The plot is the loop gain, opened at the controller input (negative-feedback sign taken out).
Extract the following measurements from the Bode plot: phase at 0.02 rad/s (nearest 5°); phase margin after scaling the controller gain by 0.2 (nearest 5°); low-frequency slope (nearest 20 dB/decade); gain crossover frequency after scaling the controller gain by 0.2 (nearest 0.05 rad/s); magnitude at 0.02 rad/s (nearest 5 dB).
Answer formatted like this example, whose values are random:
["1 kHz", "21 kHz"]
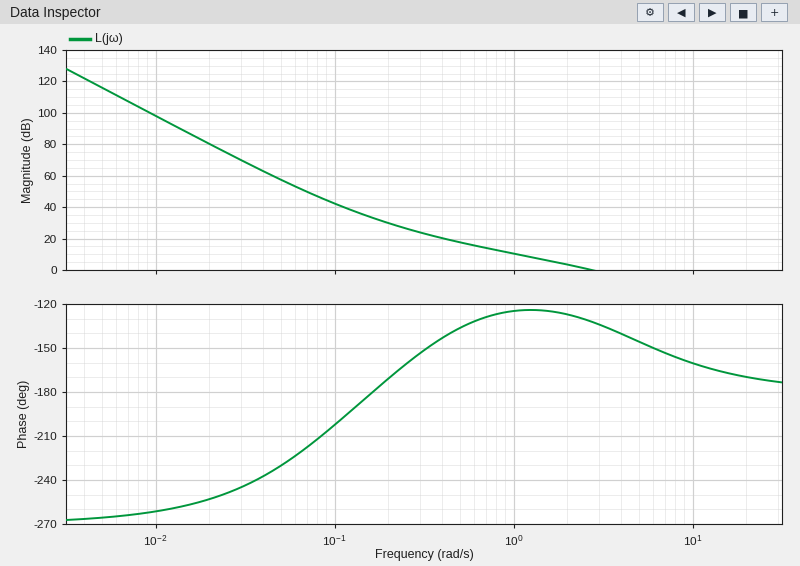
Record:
["-255°", "50°", "-60 dB/decade", "0.70 rad/s", "80 dB"]
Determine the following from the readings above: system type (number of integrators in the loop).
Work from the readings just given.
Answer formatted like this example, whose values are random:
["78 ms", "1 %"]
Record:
["3"]
